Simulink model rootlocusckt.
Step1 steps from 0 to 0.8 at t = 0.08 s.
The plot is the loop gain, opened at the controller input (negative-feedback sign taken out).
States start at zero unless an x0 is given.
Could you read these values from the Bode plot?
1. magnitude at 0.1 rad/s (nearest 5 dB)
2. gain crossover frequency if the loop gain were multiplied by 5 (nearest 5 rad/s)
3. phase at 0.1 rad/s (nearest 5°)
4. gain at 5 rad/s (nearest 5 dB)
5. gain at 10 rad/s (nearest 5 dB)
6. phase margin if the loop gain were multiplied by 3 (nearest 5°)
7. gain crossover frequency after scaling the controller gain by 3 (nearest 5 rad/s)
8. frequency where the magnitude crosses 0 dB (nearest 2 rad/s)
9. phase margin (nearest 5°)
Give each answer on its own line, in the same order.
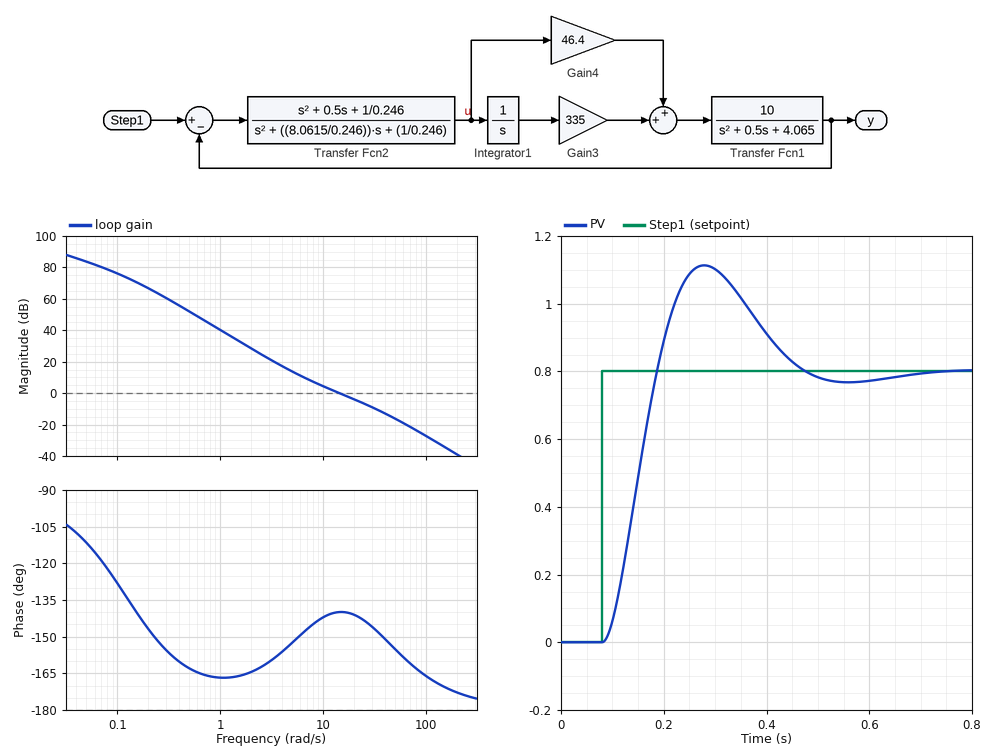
75 dB
45 rad/s
-130°
15 dB
5 dB
35°
30 rad/s
14 rad/s
40°
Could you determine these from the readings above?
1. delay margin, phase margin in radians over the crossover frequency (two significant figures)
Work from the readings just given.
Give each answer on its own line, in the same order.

0.050 s
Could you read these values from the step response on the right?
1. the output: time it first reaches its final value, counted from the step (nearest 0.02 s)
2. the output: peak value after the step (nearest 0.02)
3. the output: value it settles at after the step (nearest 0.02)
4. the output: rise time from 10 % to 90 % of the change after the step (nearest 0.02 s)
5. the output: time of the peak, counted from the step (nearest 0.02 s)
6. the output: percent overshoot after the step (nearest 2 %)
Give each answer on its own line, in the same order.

0.10 s
1.12
0.80
0.08 s
0.20 s
40 %
